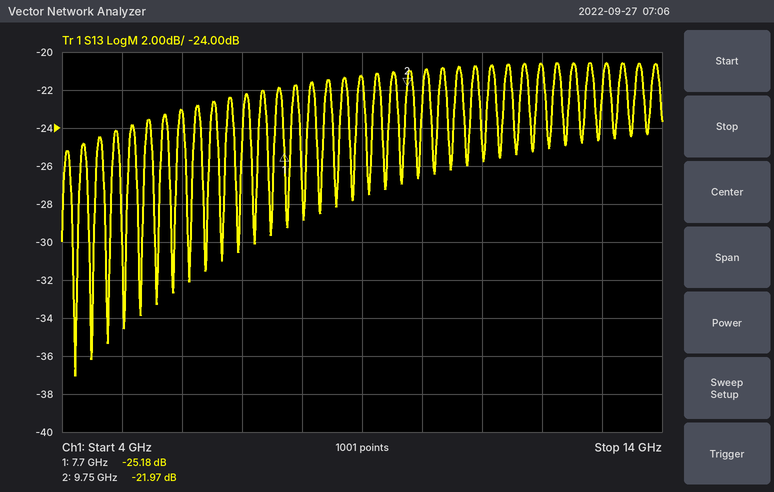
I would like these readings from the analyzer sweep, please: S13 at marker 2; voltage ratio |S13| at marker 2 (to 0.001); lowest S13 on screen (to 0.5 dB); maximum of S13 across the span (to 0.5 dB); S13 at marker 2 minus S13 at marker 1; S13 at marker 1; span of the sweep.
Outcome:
-21.97 dB
0.080
-37.0 dB
-20.5 dB
3.21 dB
-25.18 dB
10 GHz
